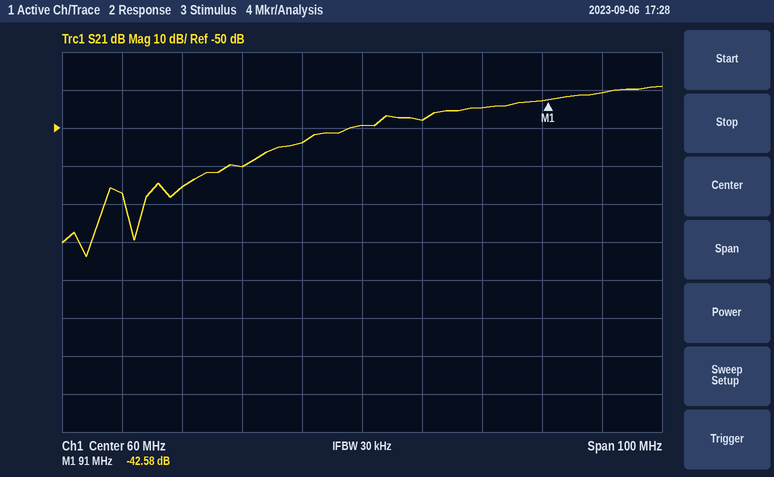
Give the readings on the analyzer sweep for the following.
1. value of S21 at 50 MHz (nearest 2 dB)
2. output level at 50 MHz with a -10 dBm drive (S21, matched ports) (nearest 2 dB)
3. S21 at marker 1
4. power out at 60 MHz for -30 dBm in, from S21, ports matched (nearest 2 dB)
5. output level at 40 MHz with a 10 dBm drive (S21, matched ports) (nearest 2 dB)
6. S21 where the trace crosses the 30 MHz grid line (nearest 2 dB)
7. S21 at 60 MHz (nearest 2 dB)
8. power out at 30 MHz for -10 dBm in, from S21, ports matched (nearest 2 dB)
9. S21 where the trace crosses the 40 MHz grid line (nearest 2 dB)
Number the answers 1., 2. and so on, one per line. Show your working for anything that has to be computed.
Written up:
1. -54 dB
2. -10 dBm + (-54 dB) = -64 dBm
3. -42.58 dB
4. -30 dBm + (-50 dB) = -80 dBm
5. 10 dBm + (-60 dB) = -50 dBm
6. -66 dB
7. -50 dB
8. -10 dBm + (-66 dB) = -76 dBm
9. -60 dB
